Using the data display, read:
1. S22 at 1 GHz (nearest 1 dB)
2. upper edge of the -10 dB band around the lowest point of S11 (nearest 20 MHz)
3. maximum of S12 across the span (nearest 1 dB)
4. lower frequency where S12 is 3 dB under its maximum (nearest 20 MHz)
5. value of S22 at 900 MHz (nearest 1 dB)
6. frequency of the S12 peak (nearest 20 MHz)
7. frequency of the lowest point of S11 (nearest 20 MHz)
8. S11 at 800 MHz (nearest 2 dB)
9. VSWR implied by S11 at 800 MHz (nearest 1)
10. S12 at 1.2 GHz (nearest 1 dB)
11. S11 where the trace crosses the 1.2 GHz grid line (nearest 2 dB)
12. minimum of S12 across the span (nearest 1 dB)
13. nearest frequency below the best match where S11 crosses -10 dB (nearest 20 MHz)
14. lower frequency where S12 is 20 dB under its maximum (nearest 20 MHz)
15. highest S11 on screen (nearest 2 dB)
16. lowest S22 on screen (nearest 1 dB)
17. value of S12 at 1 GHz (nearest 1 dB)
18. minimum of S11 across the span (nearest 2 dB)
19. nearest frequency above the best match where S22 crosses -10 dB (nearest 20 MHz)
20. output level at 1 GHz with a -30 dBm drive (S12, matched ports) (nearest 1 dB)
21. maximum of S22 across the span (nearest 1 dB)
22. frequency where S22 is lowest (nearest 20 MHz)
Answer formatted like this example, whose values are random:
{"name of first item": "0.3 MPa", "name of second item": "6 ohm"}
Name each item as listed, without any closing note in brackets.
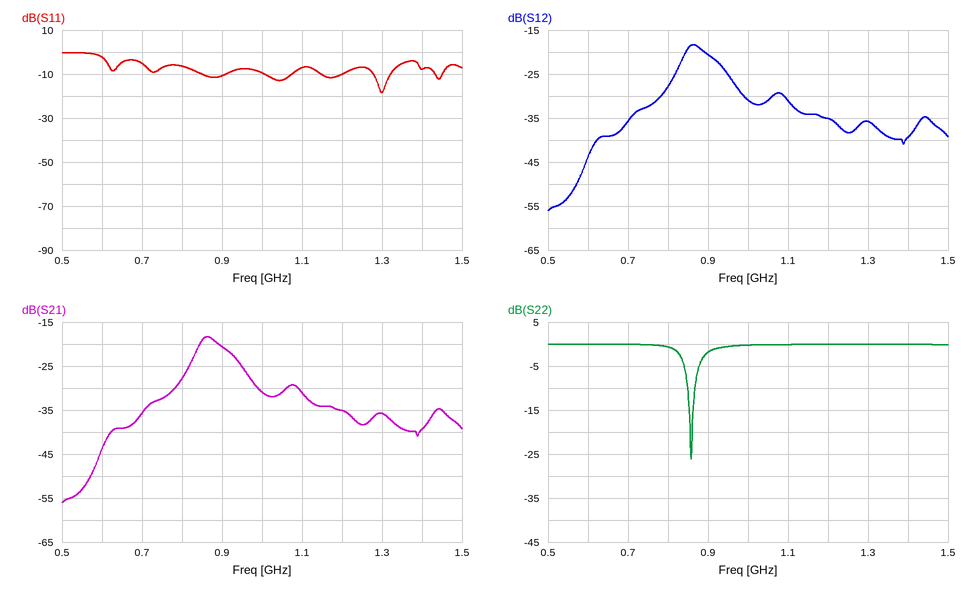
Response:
{"S22 at 1 GHz": "0 dB", "upper edge of the -10 dB band around the lowest point of S11": "1.32 GHz", "maximum of S12 across the span": "-18 dB", "lower frequency where S12 is 3 dB under its maximum": "840 MHz", "value of S22 at 900 MHz": "-2 dB", "frequency of the S12 peak": "860 MHz", "frequency of the lowest point of S11": "1.30 GHz", "S11 at 800 MHz": "-6 dB", "VSWR implied by S11 at 800 MHz": "3", "S12 at 1.2 GHz": "-35 dB", "S11 where the trace crosses the 1.2 GHz grid line": "-10 dB", "minimum of S12 across the span": "-56 dB", "nearest frequency below the best match where S11 crosses -10 dB": "1.28 GHz", "lower frequency where S12 is 20 dB under its maximum": "680 MHz", "highest S11 on screen": "0 dB", "lowest S22 on screen": "-26 dB", "value of S12 at 1 GHz": "-31 dB", "minimum of S11 across the span": "-18 dB", "nearest frequency above the best match where S22 crosses -10 dB": "860 MHz", "output level at 1 GHz with a -30 dBm drive (S12, matched ports)": "-61 dBm", "maximum of S22 across the span": "0 dB", "frequency where S22 is lowest": "860 MHz"}
